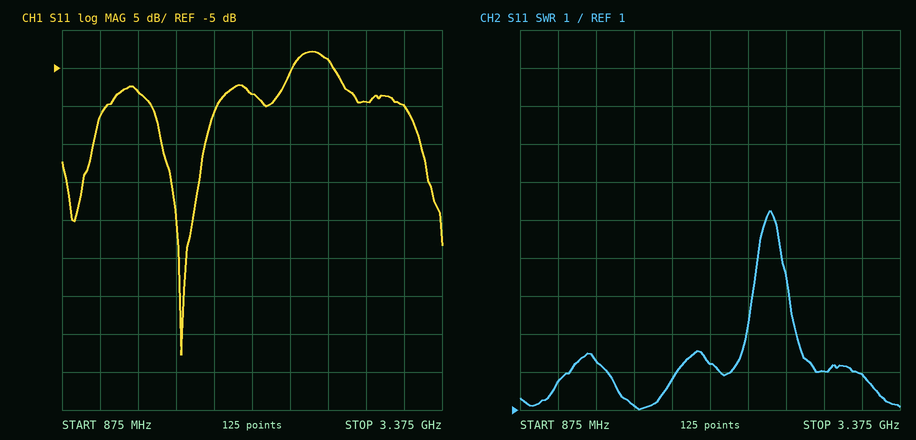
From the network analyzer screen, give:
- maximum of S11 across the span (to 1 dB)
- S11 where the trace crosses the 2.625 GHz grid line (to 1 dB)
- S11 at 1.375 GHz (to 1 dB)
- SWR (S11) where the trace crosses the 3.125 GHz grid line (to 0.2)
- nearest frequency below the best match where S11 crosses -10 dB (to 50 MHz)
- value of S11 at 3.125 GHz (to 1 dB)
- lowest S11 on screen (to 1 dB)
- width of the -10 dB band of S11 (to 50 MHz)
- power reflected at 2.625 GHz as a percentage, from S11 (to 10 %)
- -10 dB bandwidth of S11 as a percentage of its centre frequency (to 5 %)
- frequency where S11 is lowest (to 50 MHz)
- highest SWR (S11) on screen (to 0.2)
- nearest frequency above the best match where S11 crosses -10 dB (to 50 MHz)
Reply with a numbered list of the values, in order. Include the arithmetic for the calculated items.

1. -3 dB
2. -4 dB
3. -8 dB
4. 2.0
5. 1.45 GHz
6. -10 dB
7. -43 dB
8. 1.90 GHz − 1.45 GHz = 450 MHz
9. 10^(-4/10) ≈ 40 %
10. 450 MHz / 1.675 GHz ≈ 26.9 %, so 25 % to the nearest 5 %
11. 1.65 GHz
12. 6.2
13. 1.90 GHz
